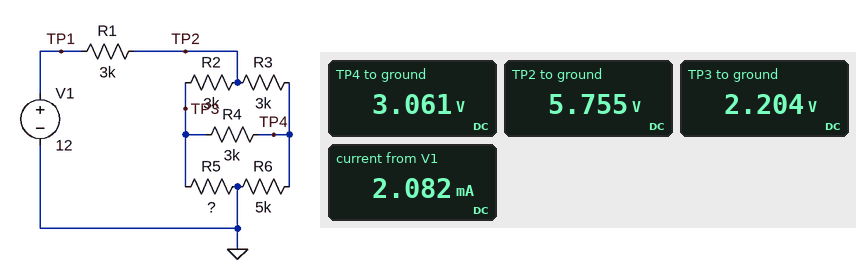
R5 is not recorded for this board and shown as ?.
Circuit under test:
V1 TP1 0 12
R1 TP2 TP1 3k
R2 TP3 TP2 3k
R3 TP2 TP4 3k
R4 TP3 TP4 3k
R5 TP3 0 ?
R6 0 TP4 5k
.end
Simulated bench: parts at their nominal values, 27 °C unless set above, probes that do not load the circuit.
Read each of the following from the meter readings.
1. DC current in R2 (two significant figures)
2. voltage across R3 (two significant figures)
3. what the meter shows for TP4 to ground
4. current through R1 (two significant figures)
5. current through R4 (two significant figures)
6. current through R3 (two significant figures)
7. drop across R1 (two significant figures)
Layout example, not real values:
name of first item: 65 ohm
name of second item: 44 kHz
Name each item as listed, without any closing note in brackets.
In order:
DC current in R2: 1.2 mA
voltage across R3: 2.7 V
what the meter shows for TP4 to ground: 3.061 V
current through R1: 2.1 mA
current through R4: 290 µA
current through R3: 900 µA
drop across R1: 6.2 V
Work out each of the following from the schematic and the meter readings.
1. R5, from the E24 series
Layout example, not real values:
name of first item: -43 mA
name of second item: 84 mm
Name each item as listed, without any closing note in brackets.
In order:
R5, from the E24 series: 1.5 kΩ
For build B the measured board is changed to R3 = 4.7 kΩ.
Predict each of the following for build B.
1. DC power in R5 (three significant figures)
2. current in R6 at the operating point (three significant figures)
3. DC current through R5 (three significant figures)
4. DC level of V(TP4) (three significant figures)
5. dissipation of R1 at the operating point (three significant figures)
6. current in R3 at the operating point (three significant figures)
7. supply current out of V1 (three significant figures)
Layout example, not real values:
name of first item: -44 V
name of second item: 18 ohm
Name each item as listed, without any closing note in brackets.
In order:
DC power in R5: 3.17 mW
current in R6 at the operating point: 538 µA
DC current through R5: 1.45 mA
DC level of V(TP4): 2.69 V
dissipation of R1 at the operating point: 11.9 mW
current in R3 at the operating point: 709 µA
supply current out of V1: 1.99 mA
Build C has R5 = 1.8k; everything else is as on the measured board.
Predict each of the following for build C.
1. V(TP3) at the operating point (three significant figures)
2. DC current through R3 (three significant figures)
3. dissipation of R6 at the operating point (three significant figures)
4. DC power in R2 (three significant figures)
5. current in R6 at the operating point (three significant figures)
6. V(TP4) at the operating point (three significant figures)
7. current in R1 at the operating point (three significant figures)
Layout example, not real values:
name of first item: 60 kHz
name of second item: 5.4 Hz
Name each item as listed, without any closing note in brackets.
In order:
V(TP3) at the operating point: 2.49 V
DC current through R3: 892 µA
dissipation of R6 at the operating point: 2.09 mW
DC power in R2: 3.89 mW
current in R6 at the operating point: 646 µA
V(TP4) at the operating point: 3.23 V
current in R1 at the operating point: 2.03 mA
